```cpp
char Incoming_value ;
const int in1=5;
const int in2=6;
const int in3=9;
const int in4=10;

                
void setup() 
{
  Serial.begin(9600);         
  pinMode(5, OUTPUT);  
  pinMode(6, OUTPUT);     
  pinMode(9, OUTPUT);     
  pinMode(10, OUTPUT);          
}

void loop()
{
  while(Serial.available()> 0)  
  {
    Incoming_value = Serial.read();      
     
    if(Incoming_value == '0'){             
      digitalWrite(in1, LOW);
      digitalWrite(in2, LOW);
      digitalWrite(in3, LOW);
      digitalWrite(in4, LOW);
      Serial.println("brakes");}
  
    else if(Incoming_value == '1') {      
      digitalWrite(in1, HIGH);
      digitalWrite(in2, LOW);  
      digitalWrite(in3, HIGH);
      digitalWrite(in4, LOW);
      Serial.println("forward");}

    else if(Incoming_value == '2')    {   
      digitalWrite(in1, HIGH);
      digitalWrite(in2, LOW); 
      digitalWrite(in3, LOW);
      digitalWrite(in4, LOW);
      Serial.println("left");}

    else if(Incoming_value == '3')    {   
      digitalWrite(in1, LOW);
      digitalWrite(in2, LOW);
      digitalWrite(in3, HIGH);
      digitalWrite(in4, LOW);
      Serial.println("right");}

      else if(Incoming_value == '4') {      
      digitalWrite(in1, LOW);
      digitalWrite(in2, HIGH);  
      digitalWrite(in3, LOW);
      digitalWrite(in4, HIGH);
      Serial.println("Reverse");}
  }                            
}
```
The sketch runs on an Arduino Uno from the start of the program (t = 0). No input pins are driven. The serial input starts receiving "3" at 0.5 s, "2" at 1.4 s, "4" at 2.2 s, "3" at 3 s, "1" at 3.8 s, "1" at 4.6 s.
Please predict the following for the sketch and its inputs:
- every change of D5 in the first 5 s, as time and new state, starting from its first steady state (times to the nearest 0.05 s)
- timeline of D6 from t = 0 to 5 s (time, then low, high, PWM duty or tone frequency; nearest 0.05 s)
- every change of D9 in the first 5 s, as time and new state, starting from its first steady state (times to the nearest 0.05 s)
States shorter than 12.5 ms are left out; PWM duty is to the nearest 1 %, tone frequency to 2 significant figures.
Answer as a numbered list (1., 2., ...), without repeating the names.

1. 0 s low; 1.4 s high; 2.2 s low; 3.8 s high
2. 0 s low; 2.2 s high; 3 s low
3. 0 s low; 0.5 s high; 1.4 s low; 3 s high
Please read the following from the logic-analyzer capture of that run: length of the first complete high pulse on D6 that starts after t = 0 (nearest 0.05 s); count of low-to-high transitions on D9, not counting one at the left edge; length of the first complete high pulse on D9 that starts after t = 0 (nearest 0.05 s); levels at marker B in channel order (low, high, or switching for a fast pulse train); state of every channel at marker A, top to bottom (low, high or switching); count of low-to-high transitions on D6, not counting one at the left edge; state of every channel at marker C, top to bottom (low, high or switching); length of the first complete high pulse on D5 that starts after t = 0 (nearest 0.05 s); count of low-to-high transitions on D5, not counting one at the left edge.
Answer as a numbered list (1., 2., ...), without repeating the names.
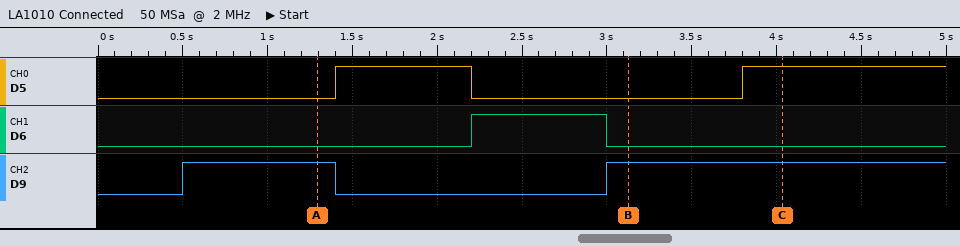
1. 0.80 s
2. 2
3. 0.90 s
4. D5 low, D6 low, D9 high
5. D5 low, D6 low, D9 high
6. 1
7. D5 high, D6 low, D9 high
8. 0.80 s
9. 2
